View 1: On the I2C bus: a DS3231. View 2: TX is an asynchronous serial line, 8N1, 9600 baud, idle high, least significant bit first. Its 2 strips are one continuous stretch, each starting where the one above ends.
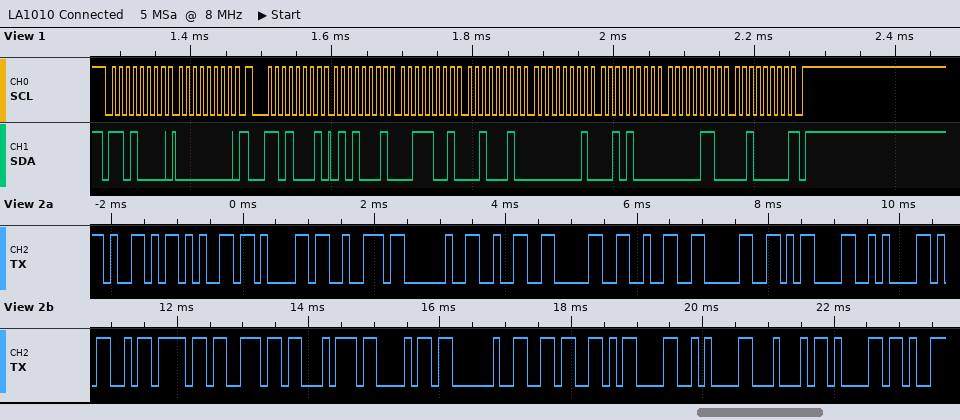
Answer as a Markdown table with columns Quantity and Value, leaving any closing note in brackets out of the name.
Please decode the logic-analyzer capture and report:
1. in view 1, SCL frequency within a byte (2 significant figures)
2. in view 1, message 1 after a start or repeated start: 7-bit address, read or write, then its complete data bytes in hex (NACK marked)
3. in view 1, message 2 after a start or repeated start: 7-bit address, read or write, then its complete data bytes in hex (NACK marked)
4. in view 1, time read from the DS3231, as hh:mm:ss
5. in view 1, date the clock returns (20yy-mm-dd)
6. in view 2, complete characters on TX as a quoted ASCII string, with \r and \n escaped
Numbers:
| Quantity | Value |
|---|---|
| in view 1, SCL frequency within a byte | 100 kHz |
| in view 1, message 1 after a start or repeated start: 7-bit address, read or write, then its complete data bytes in hex | 0x68 write: 00 |
| in view 1, message 2 after a start or repeated start: 7-bit address, read or write, then its complete data bytes in hex | 0x68 read: 51 39 22 01 28 06 20 NACK |
| in view 1, time read from the DS3231, as hh:mm:ss | 22:39:51 |
| in view 1, date the clock returns | 2020-06-28 |
| in view 2, complete characters on TX as a quoted ASCII string, with \r and \n escaped | "Year 2020\r\nMonth 6\r\nDa" |
